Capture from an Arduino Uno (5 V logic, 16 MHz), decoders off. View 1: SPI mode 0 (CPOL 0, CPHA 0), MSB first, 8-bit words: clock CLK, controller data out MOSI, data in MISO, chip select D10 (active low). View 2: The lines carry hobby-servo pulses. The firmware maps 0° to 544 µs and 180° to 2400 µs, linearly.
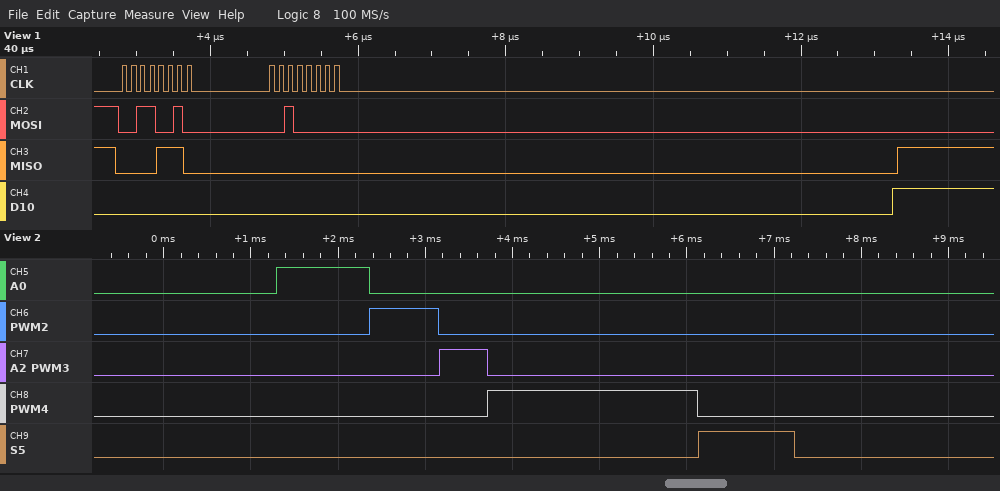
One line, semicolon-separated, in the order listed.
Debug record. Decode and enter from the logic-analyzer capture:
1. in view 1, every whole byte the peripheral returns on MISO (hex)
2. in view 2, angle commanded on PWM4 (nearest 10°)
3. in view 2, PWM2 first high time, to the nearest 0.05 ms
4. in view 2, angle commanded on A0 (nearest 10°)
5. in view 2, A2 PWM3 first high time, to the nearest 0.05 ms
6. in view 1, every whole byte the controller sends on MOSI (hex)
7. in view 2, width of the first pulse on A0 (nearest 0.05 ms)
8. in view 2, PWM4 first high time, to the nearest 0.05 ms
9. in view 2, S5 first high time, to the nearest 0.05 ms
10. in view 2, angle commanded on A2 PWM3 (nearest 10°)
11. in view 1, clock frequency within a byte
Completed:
0x0E 0x00; 180°; 0.80 ms; 50°; 0.55 ms; 0x32 0x20; 1.05 ms; 2.40 ms; 1.10 ms; 0°; 8 MHz
